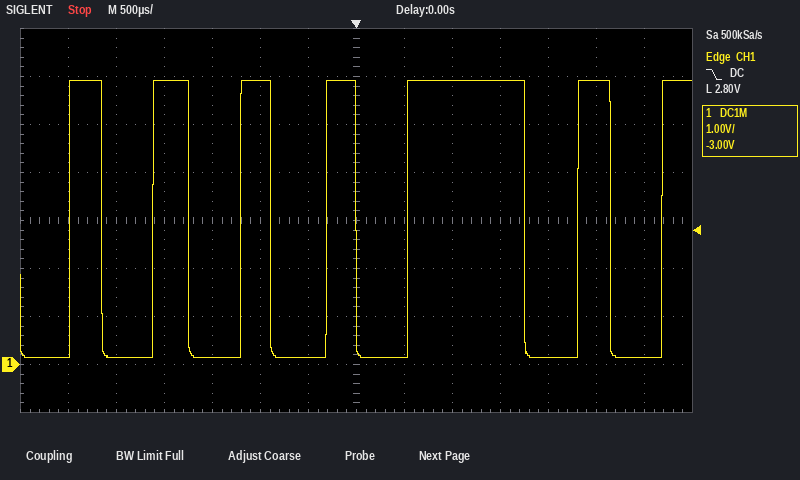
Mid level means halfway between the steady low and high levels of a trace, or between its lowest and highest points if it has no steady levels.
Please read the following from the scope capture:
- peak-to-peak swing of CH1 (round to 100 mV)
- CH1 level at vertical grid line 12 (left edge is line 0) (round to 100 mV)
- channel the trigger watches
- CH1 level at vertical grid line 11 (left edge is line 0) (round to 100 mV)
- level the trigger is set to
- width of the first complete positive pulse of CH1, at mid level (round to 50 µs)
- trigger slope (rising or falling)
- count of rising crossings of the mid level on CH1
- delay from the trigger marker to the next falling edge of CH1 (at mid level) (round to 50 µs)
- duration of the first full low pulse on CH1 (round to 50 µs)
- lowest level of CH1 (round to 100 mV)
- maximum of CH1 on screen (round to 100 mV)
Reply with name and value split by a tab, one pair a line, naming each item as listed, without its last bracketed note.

peak-to-peak swing of CH1	5.8 V
CH1 level at vertical grid line 12 (left edge is line 0)	5.9 V
channel the trigger watches	CH1
CH1 level at vertical grid line 11 (left edge is line 0)	100 mV
level the trigger is set to	2.80 V
width of the first complete positive pulse of CH1, at mid level	350 µs
trigger slope	falling
count of rising crossings of the mid level on CH1	7
delay from the trigger marker to the next falling edge of CH1 (at mid level)	1.75 ms
duration of the first full low pulse on CH1	550 µs
lowest level of CH1	100 mV
maximum of CH1 on screen	5.9 V
